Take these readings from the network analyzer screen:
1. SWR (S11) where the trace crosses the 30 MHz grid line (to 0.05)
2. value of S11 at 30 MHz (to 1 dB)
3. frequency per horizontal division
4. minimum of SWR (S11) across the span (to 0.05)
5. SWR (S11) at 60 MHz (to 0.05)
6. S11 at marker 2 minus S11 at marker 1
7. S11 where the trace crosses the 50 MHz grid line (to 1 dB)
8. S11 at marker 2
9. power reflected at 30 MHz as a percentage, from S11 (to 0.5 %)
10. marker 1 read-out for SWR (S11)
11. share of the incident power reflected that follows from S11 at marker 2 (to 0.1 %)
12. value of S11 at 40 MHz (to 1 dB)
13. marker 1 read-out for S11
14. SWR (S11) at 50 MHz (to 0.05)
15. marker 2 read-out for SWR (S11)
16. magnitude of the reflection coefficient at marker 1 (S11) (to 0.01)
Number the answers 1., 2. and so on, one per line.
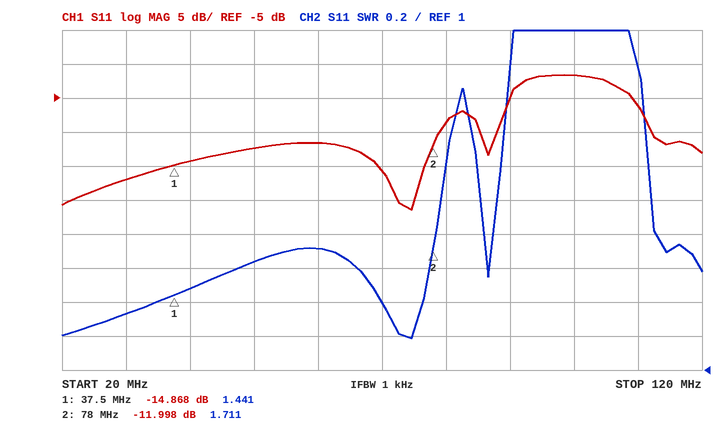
1. 1.35
2. -17 dB
3. 10 MHz
4. 1.20
5. 1.70
6. 2.870 dB
7. -12 dB
8. -11.998 dB
9. 2.0 %
10. 1.441
11. 6.3 %
12. -14 dB
13. -14.868 dB
14. 1.65
15. 1.711
16. 0.18
